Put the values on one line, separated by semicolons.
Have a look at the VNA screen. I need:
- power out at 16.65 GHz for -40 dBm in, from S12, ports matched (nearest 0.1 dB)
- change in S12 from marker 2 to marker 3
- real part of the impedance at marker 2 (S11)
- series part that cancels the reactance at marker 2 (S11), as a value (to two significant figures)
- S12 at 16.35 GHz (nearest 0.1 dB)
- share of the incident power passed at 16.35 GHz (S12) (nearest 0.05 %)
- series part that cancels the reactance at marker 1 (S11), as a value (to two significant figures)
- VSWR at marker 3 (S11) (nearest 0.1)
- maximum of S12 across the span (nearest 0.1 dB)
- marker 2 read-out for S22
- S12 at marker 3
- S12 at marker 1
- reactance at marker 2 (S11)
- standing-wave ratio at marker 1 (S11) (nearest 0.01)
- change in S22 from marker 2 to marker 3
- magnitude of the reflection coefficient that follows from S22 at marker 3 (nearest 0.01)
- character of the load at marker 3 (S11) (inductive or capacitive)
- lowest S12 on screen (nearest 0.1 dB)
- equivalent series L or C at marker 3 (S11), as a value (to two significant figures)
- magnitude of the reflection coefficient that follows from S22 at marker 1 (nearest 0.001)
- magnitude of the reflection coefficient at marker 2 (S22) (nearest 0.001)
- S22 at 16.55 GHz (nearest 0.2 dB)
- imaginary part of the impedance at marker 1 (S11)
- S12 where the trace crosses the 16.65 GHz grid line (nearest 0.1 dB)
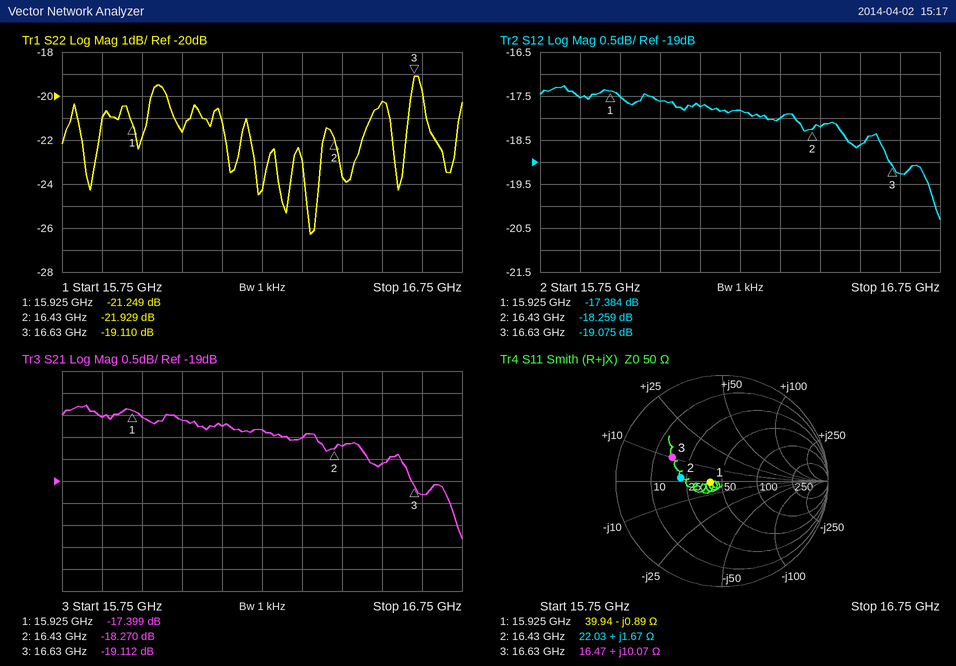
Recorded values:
-59.3 dBm; -0.816 dB; 22.03 Ω; 5.8 pF; -18.0 dB; 1.60 %; 8.9 pH; 3.2; -17.3 dB; -21.929 dB; -19.075 dB; -17.384 dB; +1.67 Ω; 1.25; 2.819 dB; 0.11; inductive; -20.3 dB; 96 pH; 0.087; 0.080; -20.2 dB; -0.89 Ω; -19.3 dB
